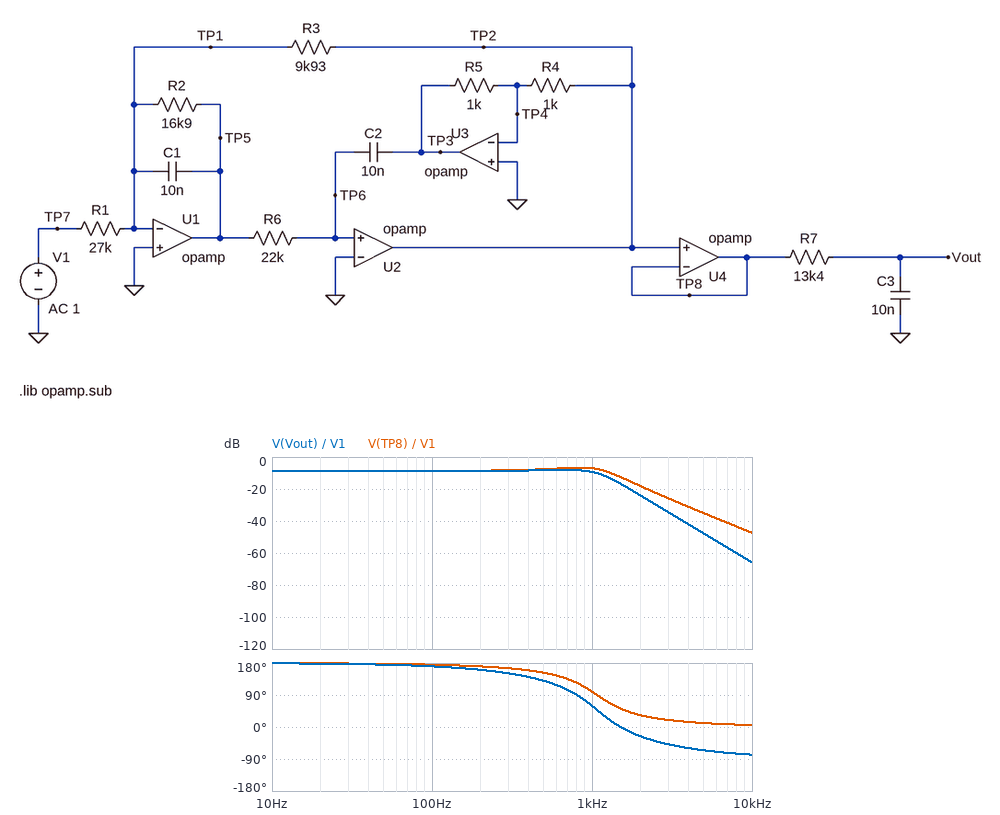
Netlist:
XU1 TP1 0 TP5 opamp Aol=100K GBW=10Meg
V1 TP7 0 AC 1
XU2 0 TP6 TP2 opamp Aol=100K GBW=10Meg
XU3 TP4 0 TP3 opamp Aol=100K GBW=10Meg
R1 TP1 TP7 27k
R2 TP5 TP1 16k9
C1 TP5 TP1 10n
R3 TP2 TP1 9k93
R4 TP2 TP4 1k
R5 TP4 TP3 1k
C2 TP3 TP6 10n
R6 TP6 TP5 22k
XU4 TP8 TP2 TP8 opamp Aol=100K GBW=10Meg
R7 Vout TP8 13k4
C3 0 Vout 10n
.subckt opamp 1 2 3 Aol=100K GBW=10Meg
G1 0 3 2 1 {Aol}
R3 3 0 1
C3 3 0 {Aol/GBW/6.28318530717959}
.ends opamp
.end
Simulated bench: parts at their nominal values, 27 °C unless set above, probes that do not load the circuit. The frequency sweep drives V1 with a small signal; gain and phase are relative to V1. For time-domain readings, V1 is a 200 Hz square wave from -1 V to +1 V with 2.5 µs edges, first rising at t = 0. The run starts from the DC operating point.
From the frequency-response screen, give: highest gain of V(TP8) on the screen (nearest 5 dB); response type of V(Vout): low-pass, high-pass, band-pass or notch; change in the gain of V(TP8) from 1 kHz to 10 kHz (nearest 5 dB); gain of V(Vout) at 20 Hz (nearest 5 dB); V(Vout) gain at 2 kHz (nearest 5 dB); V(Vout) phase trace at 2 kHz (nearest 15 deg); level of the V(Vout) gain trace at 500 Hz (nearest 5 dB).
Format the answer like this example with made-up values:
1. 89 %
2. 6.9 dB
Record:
1. -5 dB
2. low-pass
3. -40 dB
4. -10 dB
5. -25 dB
6. -30 deg
7. -10 dB
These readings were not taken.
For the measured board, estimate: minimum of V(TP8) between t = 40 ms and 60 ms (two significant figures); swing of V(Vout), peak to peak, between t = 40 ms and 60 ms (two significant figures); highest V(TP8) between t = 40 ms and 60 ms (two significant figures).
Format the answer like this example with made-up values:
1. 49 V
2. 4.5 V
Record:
1. -530 mV
2. 930 mV
3. 530 mV
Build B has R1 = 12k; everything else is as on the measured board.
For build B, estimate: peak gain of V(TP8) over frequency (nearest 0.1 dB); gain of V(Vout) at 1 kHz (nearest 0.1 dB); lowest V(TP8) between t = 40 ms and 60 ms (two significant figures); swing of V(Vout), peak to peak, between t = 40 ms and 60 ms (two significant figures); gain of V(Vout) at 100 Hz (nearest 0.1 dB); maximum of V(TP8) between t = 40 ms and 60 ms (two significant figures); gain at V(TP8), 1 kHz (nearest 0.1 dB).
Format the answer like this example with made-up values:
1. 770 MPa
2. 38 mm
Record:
1. 0.4 dB
2. -2.3 dB
3. -1.2 V
4. 2.1 V
5. -1.6 dB
6. 1.2 V
7. 0 dB
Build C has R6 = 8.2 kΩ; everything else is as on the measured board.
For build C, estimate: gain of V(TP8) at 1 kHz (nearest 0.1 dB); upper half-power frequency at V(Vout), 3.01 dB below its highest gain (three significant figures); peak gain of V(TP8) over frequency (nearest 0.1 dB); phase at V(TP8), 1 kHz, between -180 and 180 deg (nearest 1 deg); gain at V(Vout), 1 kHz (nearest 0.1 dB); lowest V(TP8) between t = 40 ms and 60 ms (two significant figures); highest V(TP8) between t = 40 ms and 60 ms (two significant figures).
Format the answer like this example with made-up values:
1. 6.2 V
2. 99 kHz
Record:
1. -6.1 dB
2. 1.95 kHz
3. -2.9 dB
4. 156 deg
5. -8.4 dB
6. -680 mV
7. 680 mV
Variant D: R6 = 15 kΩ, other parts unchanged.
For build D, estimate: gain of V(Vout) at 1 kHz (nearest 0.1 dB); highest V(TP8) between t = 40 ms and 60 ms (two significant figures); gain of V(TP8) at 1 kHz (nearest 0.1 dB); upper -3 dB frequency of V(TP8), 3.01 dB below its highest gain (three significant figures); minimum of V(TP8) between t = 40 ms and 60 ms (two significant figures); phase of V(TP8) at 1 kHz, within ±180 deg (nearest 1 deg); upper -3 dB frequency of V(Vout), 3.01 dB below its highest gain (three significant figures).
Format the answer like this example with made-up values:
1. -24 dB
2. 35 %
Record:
1. -7.8 dB
2. 590 mV
3. -5.5 dB
4. 1.55 kHz
5. -590 mV
6. 127 deg
7. 1.43 kHz
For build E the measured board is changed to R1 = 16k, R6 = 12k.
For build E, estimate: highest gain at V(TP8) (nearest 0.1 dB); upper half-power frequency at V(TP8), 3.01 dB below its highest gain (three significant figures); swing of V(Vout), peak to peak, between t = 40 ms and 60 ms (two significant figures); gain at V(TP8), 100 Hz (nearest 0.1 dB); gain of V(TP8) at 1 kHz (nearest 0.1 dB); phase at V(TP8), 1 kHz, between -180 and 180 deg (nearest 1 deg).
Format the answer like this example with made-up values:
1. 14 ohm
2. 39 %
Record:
1. 0.1 dB
2. 1.73 kHz
3. 1.6 V
4. -4.1 dB
5. -0.9 dB
6. 140 deg
